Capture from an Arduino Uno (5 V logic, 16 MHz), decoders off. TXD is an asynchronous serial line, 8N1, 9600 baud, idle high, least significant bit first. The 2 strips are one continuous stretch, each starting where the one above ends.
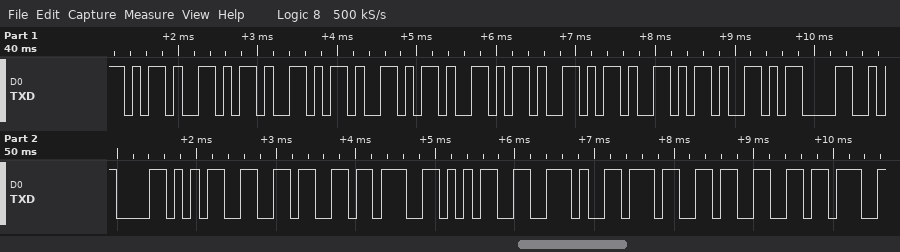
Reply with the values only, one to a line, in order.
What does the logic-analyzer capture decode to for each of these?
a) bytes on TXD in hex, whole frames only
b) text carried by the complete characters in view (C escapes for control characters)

2D 2D 2D 2D 2D 2D 2D 0D 0A 35 36 3B 35 2E 37 33 3B
"-------\r\n56;5.73;"
